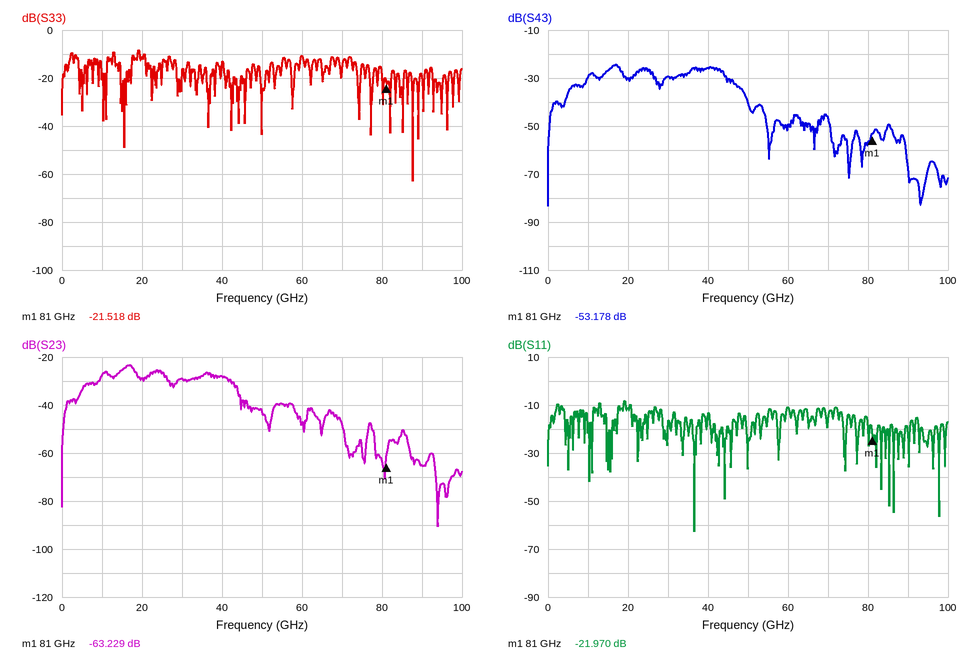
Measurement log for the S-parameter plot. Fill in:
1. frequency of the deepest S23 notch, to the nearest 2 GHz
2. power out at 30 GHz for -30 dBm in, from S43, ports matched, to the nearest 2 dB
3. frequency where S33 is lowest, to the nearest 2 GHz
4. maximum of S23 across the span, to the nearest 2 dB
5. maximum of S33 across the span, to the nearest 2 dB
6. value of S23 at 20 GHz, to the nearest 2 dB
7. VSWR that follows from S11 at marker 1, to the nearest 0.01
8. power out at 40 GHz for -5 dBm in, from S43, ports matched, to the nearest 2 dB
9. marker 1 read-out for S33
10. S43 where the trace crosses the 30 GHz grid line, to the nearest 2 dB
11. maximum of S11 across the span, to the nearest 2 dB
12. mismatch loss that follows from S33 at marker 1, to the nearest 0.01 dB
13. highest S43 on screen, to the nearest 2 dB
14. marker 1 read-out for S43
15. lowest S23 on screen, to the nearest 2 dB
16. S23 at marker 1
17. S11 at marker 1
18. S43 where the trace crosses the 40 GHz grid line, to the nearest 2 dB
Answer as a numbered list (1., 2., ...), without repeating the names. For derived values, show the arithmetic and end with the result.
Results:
1. 94 GHz
2. -30 dBm + (-30 dB) = -60 dBm
3. 88 GHz
4. -24 dB
5. -8 dB
6. -28 dB
7. (1 + 0.0797)/(1 − 0.0797) ≈ 1.17
8. -5 dBm + (-26 dB) = -30 dBm
9. -21.518 dB
10. -30 dB
11. -8 dB
12. −10 log10(1 − 10^(-21.518/10)) ≈ 0.03 dB
13. -24 dB
14. -53.178 dB
15. -90 dB
16. -63.229 dB
17. -21.970 dB
18. -26 dB
